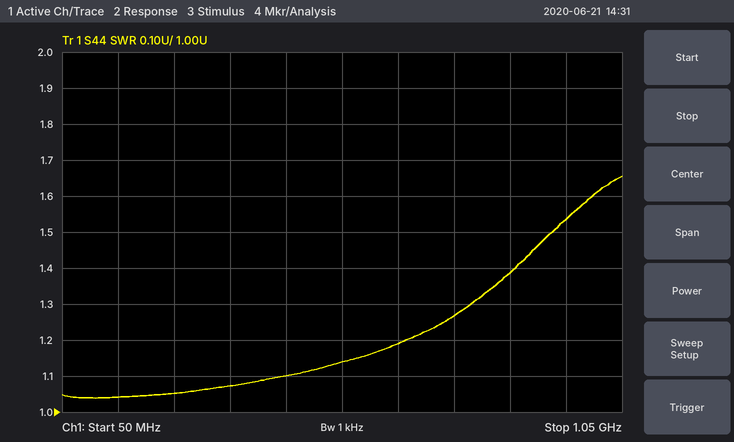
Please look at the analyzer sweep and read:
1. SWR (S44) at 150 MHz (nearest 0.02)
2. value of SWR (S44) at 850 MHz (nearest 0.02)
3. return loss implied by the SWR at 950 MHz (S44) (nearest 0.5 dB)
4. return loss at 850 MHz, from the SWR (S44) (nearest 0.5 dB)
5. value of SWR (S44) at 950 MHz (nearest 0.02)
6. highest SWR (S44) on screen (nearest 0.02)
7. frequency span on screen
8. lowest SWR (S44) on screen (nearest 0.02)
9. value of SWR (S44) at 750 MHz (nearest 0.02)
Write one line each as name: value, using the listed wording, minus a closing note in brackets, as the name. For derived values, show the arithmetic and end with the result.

SWR (S44) at 150 MHz: 1.04
value of SWR (S44) at 850 MHz: 1.38
return loss implied by the SWR at 950 MHz (S44): −20 log10((1.54 − 1)/(1.54 + 1)) ≈ 13.4 dB, so 13.5 dB to the nearest 0.5 dB
return loss at 850 MHz, from the SWR (S44): −20 log10((1.38 − 1)/(1.38 + 1)) ≈ 15.9 dB, so 16.0 dB to the nearest 0.5 dB
value of SWR (S44) at 950 MHz: 1.54
highest SWR (S44) on screen: 1.66
frequency span on screen: 1 GHz
lowest SWR (S44) on screen: 1.04
value of SWR (S44) at 750 MHz: 1.26
